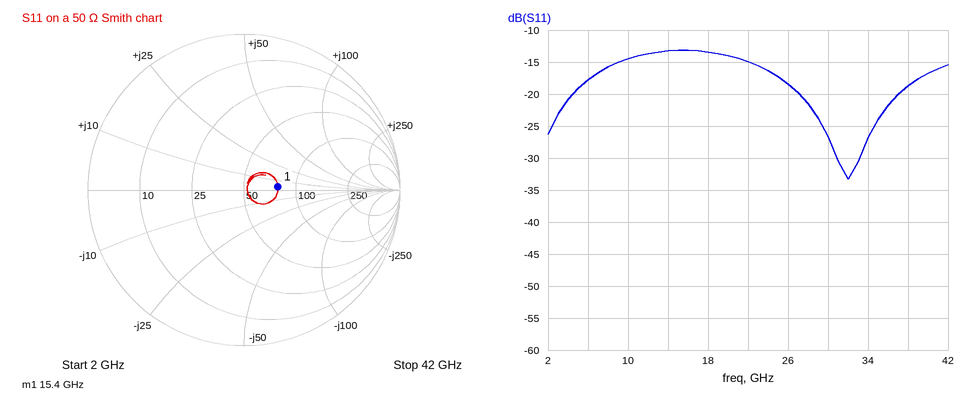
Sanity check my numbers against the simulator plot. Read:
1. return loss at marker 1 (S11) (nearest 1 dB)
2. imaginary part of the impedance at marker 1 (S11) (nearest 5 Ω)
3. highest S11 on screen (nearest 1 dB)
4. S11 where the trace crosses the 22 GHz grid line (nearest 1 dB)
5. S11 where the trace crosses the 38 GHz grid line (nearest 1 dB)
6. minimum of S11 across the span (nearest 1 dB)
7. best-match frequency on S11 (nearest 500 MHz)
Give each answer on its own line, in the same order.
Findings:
13 dB
+5 Ω
-13 dB
-15 dB
-19 dB
-33 dB
32.0 GHz
